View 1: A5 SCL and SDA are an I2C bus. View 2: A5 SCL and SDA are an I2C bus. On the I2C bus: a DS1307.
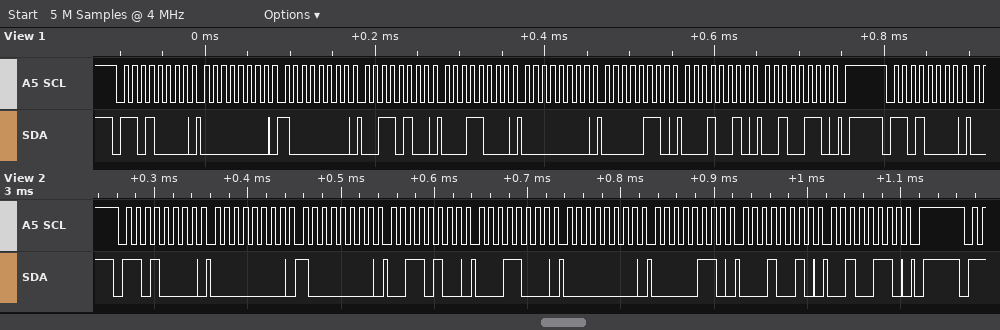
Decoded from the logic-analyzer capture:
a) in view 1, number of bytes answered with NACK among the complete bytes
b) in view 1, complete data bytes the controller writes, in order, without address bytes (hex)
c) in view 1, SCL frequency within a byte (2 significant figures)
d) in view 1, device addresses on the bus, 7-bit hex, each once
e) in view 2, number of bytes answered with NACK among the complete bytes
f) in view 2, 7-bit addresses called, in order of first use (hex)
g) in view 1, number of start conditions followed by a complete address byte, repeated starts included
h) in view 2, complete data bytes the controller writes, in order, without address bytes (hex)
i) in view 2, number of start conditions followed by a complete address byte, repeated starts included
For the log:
0
00 80 34 18 00 06 12 26
100 kHz
0x68
0
0x68
2
00 80 34 18 00 06 12 26
1
